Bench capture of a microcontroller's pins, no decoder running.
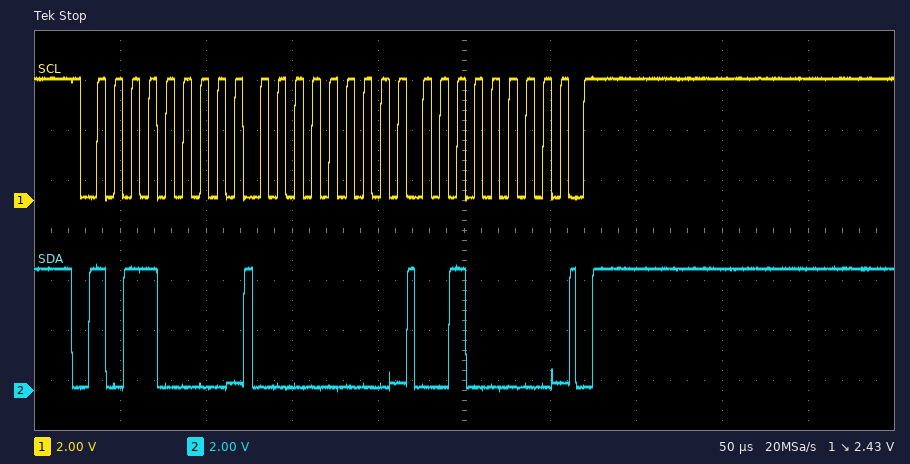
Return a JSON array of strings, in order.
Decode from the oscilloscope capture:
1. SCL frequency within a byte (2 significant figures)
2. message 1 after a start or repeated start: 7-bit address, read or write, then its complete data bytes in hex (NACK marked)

["100 kHz", "0x58 write: 00 20"]
